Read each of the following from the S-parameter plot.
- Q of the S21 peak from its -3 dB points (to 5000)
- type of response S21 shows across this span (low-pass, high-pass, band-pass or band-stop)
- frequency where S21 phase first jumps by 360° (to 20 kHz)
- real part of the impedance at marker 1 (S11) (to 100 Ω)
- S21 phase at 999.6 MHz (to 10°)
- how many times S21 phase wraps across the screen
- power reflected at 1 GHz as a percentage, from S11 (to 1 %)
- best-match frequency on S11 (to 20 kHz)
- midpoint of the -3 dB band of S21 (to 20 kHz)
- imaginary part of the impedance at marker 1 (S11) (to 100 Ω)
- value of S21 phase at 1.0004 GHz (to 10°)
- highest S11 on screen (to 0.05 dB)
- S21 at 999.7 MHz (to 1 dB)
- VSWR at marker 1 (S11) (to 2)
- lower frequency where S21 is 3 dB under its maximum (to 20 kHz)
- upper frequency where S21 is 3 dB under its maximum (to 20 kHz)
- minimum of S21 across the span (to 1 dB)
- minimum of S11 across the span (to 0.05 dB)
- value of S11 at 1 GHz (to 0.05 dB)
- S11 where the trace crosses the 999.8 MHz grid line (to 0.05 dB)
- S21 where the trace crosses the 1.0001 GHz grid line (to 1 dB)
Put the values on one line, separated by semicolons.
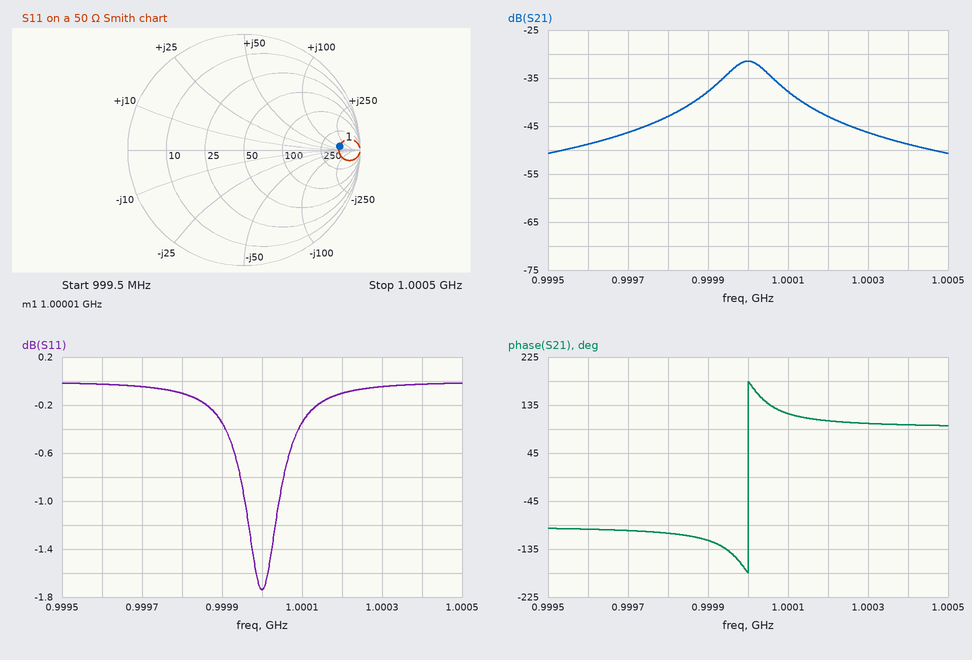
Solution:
10000; band-pass; 1.00000 GHz; 500 Ω; -100°; 1; 67 %; 1.00000 GHz; 1.00000 GHz; +100 Ω; 100°; 0.00 dB; -46 dB; 10; 999.94 MHz; 1.00006 GHz; -51 dB; -1.75 dB; -1.75 dB; -0.10 dB; -38 dB
